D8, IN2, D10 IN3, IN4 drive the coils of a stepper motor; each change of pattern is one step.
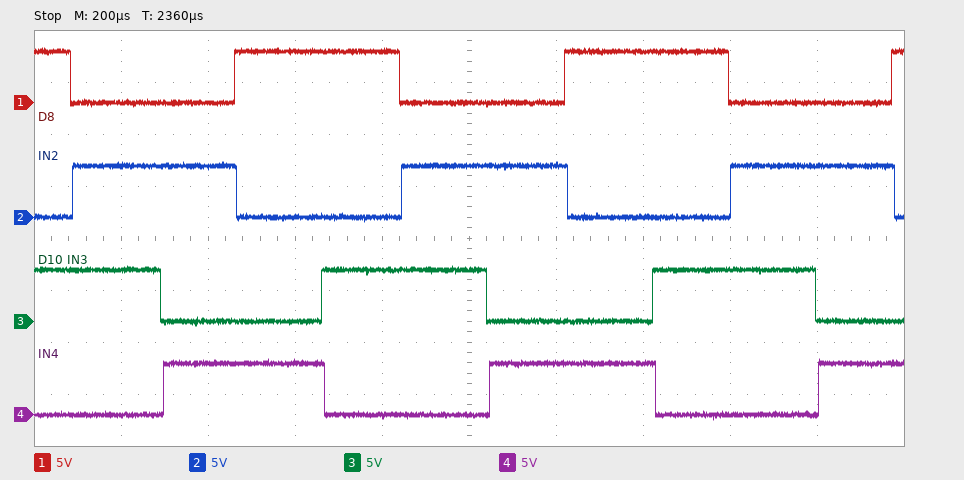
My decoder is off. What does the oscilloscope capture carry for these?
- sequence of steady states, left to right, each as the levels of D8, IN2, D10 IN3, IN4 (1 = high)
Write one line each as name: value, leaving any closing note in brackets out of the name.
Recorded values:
sequence of steady states, left to right, each as the levels of D8, IN2, D10 IN3, IN4: 1010 0110 0101 1001 1010 0110 0101 1001 1010 0110 0101 1001
